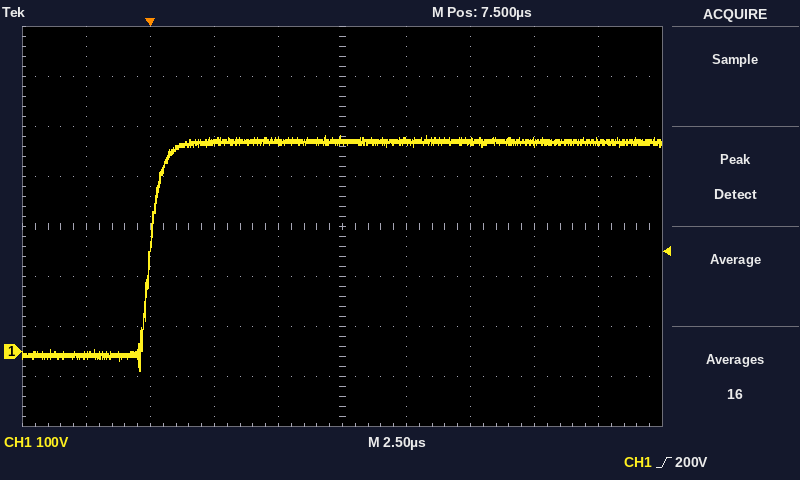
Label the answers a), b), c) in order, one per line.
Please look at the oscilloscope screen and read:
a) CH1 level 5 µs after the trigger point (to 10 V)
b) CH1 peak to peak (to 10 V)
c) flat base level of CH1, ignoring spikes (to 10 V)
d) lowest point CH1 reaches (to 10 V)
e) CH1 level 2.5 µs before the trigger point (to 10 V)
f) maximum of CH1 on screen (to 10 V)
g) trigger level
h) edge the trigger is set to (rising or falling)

a) 420 V
b) 470 V
c) -10 V
d) -40 V
e) -10 V
f) 430 V
g) 200 V
h) rising
